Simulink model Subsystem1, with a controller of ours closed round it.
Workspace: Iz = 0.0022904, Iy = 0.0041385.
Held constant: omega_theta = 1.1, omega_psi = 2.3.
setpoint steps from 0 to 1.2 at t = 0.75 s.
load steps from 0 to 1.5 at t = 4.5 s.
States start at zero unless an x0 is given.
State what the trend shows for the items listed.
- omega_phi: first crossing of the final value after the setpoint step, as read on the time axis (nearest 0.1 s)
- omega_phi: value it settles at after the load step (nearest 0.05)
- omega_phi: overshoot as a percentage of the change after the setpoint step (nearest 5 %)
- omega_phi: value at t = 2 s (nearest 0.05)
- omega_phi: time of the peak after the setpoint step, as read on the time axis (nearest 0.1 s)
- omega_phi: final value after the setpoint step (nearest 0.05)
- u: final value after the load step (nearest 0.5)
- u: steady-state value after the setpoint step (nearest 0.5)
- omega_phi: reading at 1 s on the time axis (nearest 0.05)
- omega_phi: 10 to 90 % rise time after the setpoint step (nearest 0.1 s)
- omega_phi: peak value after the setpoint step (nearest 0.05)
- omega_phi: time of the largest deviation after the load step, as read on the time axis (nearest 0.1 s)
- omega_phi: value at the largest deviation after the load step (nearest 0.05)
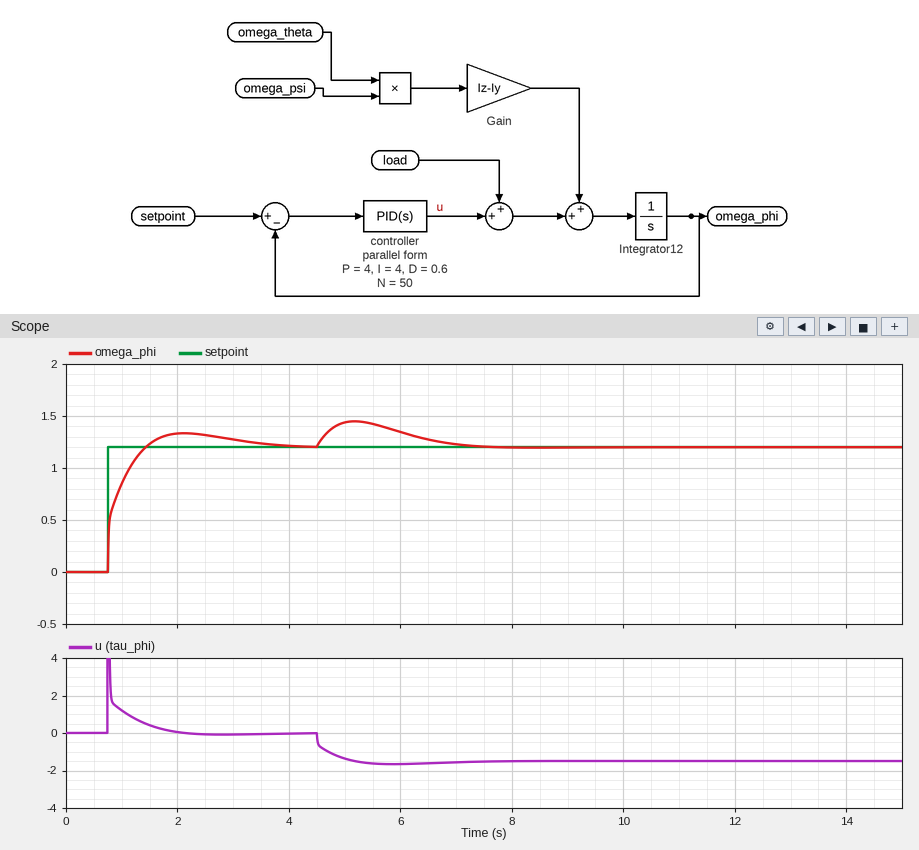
1.4 s
1.20
10 %
1.35
2.1 s
1.20
-1.5
0.0
0.85
0.5 s
1.35
5.2 s
1.45
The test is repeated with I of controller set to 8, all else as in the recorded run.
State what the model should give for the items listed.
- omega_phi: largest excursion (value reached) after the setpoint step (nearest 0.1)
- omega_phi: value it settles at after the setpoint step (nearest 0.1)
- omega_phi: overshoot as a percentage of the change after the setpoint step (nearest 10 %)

1.4
1.2
20 %
